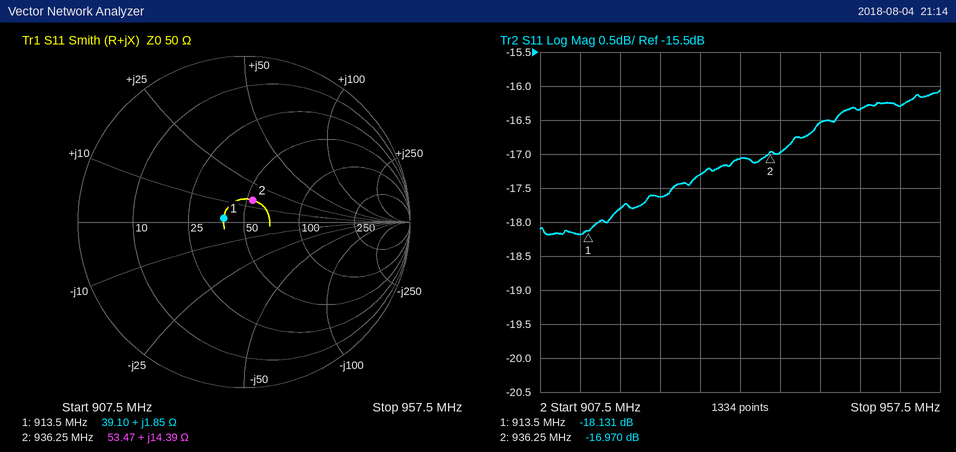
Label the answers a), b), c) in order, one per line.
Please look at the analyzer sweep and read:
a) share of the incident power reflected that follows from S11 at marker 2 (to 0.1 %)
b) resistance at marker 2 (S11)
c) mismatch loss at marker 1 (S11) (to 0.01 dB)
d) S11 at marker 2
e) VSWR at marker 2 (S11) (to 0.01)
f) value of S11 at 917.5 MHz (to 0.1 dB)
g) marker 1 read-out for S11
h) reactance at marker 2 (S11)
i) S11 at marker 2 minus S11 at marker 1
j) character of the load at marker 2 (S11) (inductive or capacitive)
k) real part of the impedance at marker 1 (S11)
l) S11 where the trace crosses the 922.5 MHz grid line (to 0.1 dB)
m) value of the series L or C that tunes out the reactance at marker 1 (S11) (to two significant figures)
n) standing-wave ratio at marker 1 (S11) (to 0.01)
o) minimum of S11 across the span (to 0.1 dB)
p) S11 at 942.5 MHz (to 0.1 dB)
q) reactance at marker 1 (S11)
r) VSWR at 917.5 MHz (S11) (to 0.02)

a) 2.0 %
b) 53.47 Ω
c) 0.07 dB
d) -16.970 dB
e) 1.33
f) -17.8 dB
g) -18.131 dB
h) +14.39 Ω
i) 1.161 dB
j) inductive
k) 39.10 Ω
l) -17.6 dB
m) 94 pF
n) 1.28
o) -18.2 dB
p) -16.5 dB
q) +1.85 Ω
r) 1.30
